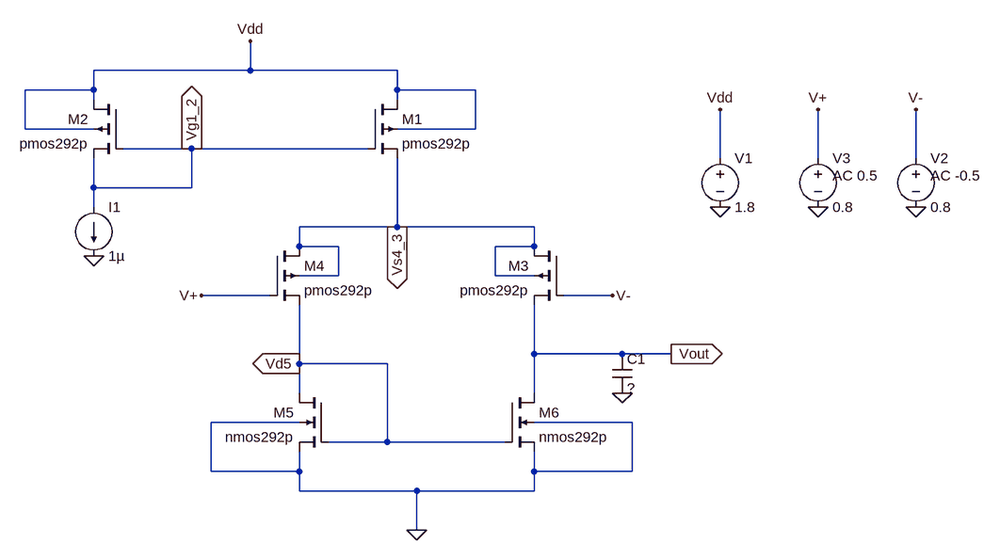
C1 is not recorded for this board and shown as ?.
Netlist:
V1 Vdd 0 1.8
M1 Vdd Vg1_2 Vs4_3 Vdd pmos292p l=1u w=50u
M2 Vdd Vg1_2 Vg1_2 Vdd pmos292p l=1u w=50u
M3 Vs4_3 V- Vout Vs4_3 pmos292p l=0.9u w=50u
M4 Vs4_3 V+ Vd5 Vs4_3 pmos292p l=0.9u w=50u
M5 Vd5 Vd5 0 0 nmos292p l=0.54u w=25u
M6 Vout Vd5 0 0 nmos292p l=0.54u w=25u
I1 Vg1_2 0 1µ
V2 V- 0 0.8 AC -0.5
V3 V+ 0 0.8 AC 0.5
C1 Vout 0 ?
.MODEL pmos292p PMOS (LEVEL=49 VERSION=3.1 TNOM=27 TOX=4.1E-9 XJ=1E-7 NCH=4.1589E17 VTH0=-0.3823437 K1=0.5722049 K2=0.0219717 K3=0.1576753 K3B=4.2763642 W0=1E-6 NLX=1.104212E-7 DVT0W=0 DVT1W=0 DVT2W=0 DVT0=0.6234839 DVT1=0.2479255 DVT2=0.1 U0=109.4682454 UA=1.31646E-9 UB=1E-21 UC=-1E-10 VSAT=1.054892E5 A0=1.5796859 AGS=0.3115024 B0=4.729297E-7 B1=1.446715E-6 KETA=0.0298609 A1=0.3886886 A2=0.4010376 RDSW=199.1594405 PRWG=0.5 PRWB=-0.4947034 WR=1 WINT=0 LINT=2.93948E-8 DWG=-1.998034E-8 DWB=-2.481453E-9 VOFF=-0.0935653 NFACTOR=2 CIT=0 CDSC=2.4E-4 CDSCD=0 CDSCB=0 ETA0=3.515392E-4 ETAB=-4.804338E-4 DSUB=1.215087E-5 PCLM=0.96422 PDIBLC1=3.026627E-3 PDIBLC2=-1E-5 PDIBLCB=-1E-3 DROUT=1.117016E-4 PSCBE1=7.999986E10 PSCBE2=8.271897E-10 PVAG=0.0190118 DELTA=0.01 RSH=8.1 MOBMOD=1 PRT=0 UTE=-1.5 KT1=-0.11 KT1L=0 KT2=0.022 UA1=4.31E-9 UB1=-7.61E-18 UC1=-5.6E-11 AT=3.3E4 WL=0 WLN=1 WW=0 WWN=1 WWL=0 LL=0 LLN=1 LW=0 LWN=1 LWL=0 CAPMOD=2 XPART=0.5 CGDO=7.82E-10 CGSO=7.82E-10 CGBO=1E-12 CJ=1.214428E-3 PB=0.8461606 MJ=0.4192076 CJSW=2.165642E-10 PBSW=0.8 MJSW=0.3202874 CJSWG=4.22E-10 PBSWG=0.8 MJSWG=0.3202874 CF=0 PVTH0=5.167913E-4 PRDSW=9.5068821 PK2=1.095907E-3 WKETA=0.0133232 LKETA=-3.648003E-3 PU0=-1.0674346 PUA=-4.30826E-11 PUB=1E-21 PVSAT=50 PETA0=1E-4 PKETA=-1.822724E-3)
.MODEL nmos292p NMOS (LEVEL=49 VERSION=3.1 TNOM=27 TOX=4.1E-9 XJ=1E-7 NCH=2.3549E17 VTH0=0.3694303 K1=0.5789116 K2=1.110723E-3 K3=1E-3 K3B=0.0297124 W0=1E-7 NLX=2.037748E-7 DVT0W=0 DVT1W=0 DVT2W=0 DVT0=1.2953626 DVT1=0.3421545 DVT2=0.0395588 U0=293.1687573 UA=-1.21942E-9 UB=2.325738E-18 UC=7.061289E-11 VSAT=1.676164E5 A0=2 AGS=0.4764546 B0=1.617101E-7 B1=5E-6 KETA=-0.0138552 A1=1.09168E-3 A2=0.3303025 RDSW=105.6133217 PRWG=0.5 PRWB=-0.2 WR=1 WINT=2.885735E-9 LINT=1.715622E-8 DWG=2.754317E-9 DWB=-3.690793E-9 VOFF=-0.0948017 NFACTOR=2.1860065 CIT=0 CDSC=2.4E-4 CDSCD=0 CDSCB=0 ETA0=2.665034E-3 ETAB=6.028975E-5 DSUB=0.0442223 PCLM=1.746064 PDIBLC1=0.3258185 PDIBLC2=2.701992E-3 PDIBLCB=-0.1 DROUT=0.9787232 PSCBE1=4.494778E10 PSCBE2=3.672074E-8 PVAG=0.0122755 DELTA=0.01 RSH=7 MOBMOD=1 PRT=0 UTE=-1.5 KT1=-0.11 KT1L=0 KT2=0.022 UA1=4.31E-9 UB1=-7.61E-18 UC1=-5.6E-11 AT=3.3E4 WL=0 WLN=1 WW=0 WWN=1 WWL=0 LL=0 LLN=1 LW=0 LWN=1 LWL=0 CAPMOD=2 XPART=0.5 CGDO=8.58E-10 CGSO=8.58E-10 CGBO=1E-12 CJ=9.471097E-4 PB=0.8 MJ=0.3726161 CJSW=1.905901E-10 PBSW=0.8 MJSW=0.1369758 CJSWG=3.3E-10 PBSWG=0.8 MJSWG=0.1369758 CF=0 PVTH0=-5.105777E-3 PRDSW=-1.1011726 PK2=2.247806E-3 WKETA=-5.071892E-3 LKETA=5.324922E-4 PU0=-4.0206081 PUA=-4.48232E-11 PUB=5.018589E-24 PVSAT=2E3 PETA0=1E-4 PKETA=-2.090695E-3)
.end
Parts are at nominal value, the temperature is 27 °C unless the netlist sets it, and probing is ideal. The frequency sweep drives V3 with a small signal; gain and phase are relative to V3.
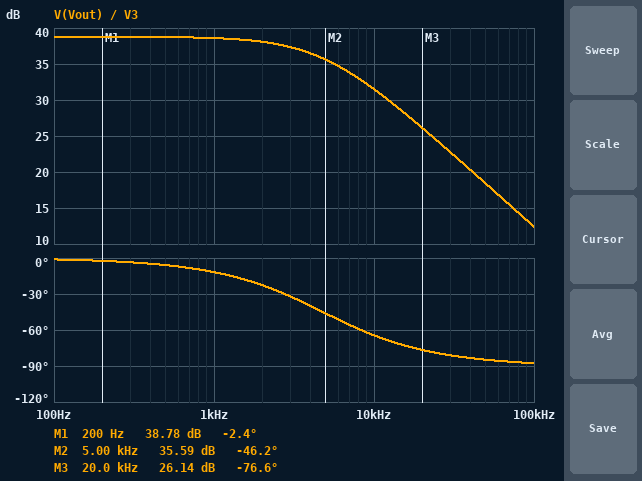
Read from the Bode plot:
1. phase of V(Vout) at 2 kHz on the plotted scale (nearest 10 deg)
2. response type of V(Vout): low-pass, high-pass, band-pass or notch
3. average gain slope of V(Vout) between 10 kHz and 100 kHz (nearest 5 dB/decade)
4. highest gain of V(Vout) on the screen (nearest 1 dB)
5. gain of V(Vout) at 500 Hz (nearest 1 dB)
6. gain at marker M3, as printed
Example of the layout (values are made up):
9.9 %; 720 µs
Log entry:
-20 deg; low-pass; -20 dB/decade; 39 dB; 39 dB; 26.14 dB
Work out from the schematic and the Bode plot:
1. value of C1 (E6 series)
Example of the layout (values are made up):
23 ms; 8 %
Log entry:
6.8 pF
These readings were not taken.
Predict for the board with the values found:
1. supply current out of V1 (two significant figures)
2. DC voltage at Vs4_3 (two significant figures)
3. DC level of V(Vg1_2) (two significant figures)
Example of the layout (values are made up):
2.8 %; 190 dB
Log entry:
2.0 µA; 1.1 V; 1.4 V
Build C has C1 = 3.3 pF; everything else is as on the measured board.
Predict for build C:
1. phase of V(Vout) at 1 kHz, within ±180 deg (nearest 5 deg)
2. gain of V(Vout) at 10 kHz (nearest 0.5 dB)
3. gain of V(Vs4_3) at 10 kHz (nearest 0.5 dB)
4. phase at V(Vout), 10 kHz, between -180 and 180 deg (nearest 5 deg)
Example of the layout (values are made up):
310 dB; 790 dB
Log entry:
-5 deg; 35.5 dB; -8.0 dB; -45 deg
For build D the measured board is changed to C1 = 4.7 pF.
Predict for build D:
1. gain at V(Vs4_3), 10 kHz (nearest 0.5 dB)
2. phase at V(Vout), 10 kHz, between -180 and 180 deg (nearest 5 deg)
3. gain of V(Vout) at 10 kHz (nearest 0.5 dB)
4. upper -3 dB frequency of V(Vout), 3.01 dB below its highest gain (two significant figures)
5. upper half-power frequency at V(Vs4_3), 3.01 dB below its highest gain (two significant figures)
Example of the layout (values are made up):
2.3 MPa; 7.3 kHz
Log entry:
-9.0 dB; -55 deg; 34.0 dB; 6.9 kHz; 9.5 kHz
